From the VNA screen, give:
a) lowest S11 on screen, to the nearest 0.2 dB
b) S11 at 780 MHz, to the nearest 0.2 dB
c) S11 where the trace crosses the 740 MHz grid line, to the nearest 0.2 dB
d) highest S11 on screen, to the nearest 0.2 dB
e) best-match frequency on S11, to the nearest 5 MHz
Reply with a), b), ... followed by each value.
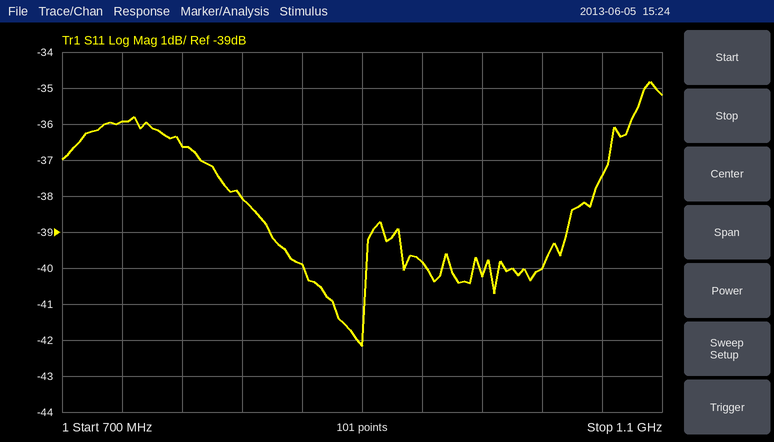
a) -42.2 dB
b) -36.6 dB
c) -36.0 dB
d) -34.8 dB
e) 900 MHz
